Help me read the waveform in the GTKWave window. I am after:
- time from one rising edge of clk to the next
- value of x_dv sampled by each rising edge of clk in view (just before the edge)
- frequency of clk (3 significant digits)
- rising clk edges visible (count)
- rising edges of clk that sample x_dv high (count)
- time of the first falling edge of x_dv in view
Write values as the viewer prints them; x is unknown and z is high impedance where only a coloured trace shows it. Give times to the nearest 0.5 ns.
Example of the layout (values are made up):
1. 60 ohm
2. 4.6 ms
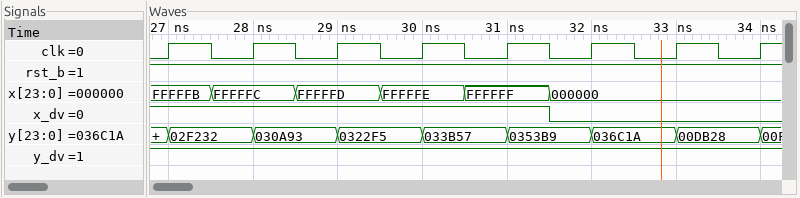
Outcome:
1. 1 ns
2. 1 1 1 1 1 0 0 0
3. 1.00 GHz
4. 8
5. 5
6. 31.5 ns
